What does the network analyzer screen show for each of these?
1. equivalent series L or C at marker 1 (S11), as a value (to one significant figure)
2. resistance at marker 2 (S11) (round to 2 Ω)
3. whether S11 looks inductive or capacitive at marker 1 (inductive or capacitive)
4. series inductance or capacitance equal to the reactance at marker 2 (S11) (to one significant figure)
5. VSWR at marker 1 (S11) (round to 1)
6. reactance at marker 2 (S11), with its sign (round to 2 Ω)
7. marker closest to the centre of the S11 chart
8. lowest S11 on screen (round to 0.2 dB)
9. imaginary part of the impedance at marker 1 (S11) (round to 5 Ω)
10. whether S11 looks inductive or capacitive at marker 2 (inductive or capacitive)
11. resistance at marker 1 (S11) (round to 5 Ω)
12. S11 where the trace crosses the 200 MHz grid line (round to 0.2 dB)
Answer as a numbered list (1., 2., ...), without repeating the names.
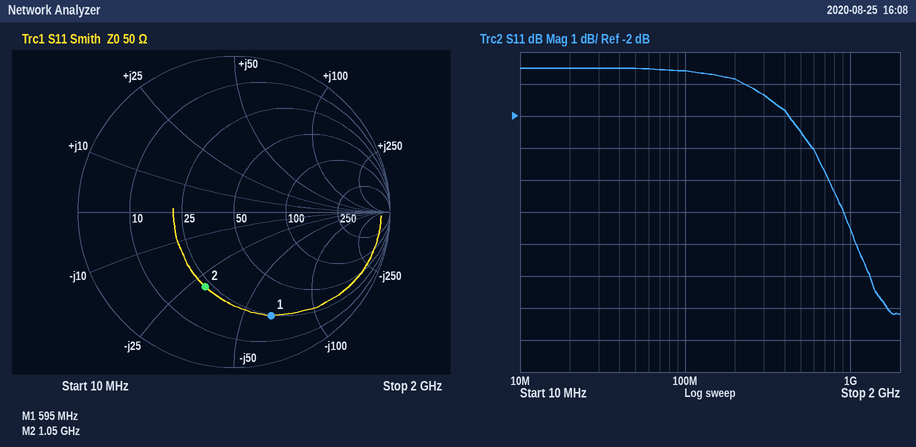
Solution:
1. 4 pF
2. 22 Ω
3. capacitive
4. 5 pF
5. 6
6. -30 Ω
7. marker 2
8. -8.2 dB
9. -65 Ω
10. capacitive
11. 25 Ω
12. -0.8 dB
